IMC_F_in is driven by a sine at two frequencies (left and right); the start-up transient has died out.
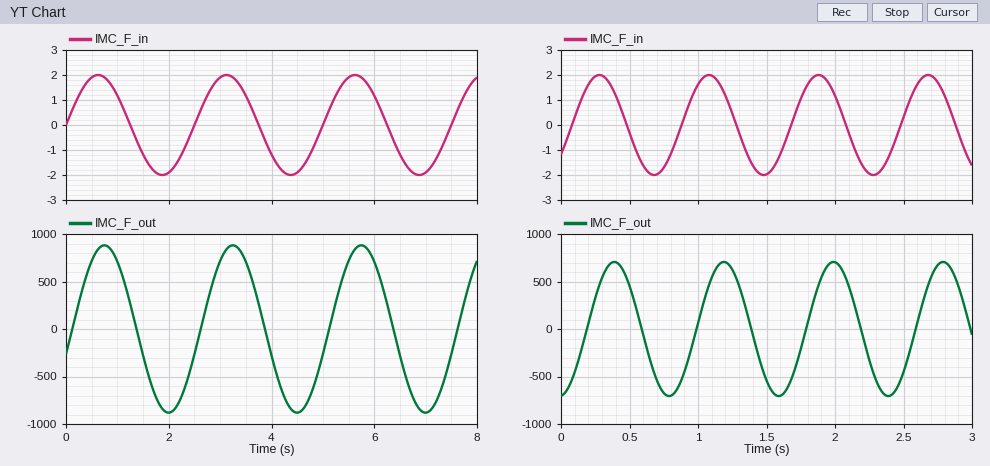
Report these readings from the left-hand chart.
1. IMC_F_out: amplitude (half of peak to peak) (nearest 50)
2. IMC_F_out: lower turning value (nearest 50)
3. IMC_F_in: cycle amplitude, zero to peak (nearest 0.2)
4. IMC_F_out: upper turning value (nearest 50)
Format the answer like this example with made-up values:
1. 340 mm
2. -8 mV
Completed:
1. 900
2. -900
3. 2.0
4. 900
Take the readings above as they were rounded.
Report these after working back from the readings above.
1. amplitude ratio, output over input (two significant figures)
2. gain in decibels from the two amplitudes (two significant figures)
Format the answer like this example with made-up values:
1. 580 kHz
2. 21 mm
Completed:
1. 450
2. 53 dB
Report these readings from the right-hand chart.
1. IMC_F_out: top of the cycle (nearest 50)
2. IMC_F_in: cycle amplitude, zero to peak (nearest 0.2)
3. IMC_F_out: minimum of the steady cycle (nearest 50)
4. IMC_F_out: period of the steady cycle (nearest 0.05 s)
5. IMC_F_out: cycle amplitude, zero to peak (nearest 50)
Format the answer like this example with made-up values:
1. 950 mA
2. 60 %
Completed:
1. 700
2. 2.0
3. -700
4. 0.80 s
5. 700
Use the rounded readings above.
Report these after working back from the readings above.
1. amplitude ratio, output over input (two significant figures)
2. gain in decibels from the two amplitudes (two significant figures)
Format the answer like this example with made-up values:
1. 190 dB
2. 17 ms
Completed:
1. 350
2. 51 dB
